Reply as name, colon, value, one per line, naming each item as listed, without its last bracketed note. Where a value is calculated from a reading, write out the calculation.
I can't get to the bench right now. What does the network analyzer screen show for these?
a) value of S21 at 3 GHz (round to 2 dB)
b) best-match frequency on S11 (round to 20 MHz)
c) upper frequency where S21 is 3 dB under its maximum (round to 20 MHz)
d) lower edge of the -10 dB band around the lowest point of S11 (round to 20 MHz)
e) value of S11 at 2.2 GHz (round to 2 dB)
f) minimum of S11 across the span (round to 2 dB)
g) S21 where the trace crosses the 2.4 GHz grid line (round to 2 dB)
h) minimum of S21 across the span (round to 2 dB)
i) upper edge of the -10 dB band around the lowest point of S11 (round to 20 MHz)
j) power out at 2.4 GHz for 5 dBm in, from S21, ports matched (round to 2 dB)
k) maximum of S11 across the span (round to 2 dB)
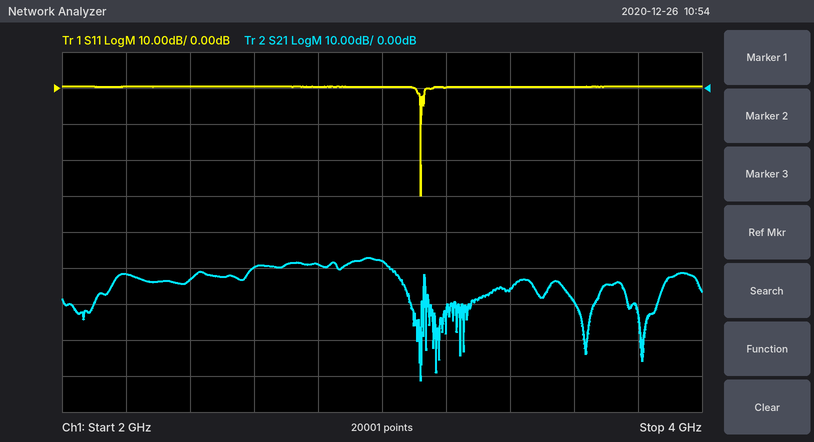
value of S21 at 3 GHz: -48 dB
best-match frequency on S11: 3.12 GHz
upper frequency where S21 is 3 dB under its maximum: 3.02 GHz
lower edge of the -10 dB band around the lowest point of S11: 3.12 GHz
value of S11 at 2.2 GHz: 0 dB
minimum of S11 across the span: -30 dB
S21 where the trace crosses the 2.4 GHz grid line: -54 dB
minimum of S21 across the span: -82 dB
upper edge of the -10 dB band around the lowest point of S11: 3.12 GHz
power out at 2.4 GHz for 5 dBm in, from S21, ports matched: 5 dBm + (-54 dB) = -48 dBm
maximum of S11 across the span: 0 dB
